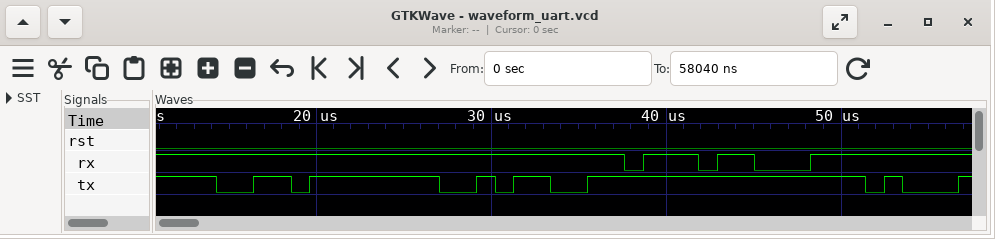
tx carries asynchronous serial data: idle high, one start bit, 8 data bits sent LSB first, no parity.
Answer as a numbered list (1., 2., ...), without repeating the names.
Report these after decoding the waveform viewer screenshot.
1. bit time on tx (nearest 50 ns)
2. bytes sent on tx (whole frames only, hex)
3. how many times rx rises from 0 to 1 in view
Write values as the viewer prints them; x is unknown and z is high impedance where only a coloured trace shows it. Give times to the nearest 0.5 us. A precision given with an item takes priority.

1. 1050 ns
2. F6, 9A
3. 3
